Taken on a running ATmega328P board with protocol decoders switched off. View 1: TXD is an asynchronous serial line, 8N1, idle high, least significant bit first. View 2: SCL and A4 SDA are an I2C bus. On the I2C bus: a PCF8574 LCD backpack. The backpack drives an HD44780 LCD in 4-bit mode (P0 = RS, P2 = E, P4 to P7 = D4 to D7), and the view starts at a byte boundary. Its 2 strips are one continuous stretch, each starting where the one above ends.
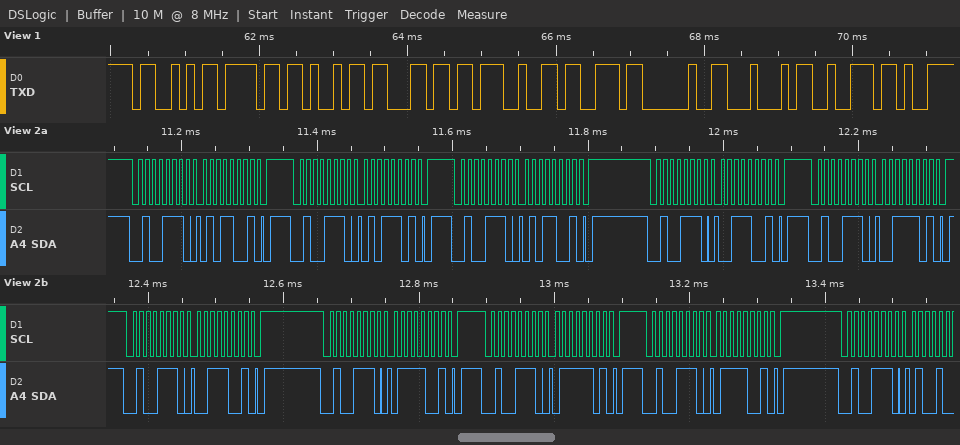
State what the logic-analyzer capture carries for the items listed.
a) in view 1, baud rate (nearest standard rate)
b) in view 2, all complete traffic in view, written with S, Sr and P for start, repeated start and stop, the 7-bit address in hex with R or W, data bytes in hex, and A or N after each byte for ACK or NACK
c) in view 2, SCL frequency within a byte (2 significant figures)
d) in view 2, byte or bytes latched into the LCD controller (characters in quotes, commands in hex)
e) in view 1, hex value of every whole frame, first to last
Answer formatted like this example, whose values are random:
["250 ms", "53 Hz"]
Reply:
["9600 baud", "S 27W A 59 A P S 27W A 5D A P S 27W A 59 A P S 27W A 39 A P S 27W A 3D A P S 27W A 39 A P S 27W A 79 A P S 27W A 7D A P S 27W A 79 A P S 27W A", "100 kHz", "'S'", "53 6F 69 6C 27 73 20 44 72"]
